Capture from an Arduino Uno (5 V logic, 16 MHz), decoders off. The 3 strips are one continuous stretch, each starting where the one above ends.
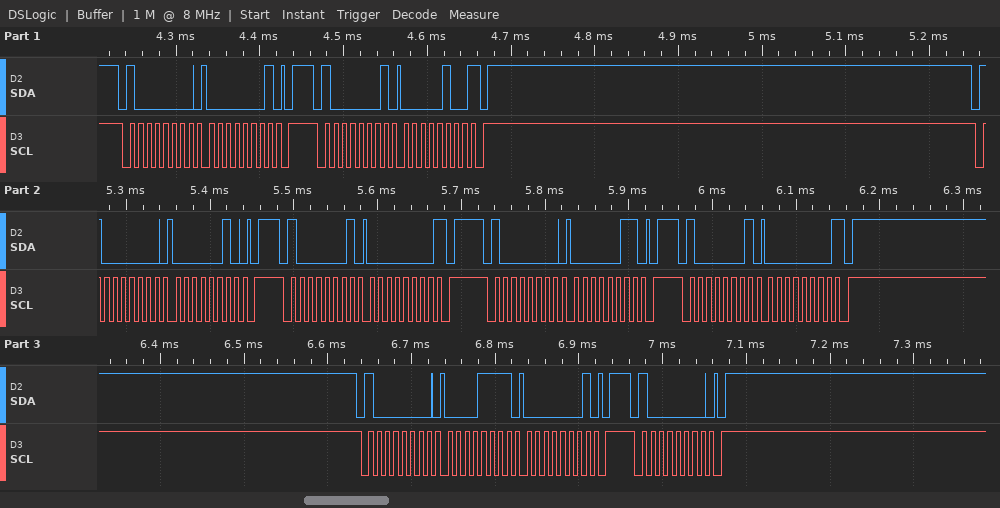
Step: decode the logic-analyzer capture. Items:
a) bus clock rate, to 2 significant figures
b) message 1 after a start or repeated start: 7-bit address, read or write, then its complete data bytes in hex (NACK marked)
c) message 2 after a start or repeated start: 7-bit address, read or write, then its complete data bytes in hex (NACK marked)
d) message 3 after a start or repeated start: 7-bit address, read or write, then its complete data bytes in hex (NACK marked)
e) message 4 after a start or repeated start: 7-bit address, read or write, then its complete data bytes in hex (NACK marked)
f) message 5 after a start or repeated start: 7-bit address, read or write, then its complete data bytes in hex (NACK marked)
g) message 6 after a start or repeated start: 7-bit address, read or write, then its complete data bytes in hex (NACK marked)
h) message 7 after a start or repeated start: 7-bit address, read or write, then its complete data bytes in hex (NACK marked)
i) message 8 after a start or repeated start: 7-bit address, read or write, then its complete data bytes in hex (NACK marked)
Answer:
100 kHz
0x40 write: 01
0x40 read: 04 NACK
0x40 write: 02
0x40 read: 00 NACK
0x40 write: 03
0x40 read: 00 NACK
0x40 write: 0F 01
0x40 write
